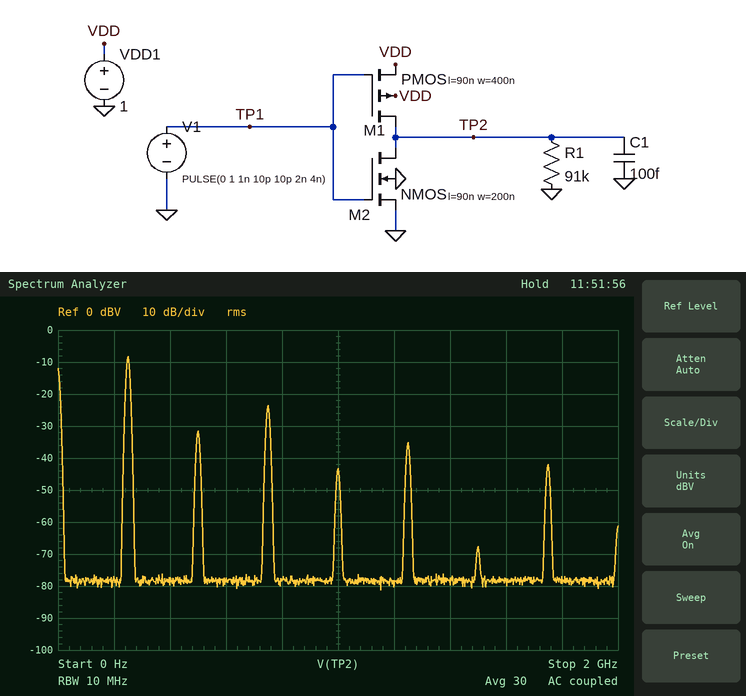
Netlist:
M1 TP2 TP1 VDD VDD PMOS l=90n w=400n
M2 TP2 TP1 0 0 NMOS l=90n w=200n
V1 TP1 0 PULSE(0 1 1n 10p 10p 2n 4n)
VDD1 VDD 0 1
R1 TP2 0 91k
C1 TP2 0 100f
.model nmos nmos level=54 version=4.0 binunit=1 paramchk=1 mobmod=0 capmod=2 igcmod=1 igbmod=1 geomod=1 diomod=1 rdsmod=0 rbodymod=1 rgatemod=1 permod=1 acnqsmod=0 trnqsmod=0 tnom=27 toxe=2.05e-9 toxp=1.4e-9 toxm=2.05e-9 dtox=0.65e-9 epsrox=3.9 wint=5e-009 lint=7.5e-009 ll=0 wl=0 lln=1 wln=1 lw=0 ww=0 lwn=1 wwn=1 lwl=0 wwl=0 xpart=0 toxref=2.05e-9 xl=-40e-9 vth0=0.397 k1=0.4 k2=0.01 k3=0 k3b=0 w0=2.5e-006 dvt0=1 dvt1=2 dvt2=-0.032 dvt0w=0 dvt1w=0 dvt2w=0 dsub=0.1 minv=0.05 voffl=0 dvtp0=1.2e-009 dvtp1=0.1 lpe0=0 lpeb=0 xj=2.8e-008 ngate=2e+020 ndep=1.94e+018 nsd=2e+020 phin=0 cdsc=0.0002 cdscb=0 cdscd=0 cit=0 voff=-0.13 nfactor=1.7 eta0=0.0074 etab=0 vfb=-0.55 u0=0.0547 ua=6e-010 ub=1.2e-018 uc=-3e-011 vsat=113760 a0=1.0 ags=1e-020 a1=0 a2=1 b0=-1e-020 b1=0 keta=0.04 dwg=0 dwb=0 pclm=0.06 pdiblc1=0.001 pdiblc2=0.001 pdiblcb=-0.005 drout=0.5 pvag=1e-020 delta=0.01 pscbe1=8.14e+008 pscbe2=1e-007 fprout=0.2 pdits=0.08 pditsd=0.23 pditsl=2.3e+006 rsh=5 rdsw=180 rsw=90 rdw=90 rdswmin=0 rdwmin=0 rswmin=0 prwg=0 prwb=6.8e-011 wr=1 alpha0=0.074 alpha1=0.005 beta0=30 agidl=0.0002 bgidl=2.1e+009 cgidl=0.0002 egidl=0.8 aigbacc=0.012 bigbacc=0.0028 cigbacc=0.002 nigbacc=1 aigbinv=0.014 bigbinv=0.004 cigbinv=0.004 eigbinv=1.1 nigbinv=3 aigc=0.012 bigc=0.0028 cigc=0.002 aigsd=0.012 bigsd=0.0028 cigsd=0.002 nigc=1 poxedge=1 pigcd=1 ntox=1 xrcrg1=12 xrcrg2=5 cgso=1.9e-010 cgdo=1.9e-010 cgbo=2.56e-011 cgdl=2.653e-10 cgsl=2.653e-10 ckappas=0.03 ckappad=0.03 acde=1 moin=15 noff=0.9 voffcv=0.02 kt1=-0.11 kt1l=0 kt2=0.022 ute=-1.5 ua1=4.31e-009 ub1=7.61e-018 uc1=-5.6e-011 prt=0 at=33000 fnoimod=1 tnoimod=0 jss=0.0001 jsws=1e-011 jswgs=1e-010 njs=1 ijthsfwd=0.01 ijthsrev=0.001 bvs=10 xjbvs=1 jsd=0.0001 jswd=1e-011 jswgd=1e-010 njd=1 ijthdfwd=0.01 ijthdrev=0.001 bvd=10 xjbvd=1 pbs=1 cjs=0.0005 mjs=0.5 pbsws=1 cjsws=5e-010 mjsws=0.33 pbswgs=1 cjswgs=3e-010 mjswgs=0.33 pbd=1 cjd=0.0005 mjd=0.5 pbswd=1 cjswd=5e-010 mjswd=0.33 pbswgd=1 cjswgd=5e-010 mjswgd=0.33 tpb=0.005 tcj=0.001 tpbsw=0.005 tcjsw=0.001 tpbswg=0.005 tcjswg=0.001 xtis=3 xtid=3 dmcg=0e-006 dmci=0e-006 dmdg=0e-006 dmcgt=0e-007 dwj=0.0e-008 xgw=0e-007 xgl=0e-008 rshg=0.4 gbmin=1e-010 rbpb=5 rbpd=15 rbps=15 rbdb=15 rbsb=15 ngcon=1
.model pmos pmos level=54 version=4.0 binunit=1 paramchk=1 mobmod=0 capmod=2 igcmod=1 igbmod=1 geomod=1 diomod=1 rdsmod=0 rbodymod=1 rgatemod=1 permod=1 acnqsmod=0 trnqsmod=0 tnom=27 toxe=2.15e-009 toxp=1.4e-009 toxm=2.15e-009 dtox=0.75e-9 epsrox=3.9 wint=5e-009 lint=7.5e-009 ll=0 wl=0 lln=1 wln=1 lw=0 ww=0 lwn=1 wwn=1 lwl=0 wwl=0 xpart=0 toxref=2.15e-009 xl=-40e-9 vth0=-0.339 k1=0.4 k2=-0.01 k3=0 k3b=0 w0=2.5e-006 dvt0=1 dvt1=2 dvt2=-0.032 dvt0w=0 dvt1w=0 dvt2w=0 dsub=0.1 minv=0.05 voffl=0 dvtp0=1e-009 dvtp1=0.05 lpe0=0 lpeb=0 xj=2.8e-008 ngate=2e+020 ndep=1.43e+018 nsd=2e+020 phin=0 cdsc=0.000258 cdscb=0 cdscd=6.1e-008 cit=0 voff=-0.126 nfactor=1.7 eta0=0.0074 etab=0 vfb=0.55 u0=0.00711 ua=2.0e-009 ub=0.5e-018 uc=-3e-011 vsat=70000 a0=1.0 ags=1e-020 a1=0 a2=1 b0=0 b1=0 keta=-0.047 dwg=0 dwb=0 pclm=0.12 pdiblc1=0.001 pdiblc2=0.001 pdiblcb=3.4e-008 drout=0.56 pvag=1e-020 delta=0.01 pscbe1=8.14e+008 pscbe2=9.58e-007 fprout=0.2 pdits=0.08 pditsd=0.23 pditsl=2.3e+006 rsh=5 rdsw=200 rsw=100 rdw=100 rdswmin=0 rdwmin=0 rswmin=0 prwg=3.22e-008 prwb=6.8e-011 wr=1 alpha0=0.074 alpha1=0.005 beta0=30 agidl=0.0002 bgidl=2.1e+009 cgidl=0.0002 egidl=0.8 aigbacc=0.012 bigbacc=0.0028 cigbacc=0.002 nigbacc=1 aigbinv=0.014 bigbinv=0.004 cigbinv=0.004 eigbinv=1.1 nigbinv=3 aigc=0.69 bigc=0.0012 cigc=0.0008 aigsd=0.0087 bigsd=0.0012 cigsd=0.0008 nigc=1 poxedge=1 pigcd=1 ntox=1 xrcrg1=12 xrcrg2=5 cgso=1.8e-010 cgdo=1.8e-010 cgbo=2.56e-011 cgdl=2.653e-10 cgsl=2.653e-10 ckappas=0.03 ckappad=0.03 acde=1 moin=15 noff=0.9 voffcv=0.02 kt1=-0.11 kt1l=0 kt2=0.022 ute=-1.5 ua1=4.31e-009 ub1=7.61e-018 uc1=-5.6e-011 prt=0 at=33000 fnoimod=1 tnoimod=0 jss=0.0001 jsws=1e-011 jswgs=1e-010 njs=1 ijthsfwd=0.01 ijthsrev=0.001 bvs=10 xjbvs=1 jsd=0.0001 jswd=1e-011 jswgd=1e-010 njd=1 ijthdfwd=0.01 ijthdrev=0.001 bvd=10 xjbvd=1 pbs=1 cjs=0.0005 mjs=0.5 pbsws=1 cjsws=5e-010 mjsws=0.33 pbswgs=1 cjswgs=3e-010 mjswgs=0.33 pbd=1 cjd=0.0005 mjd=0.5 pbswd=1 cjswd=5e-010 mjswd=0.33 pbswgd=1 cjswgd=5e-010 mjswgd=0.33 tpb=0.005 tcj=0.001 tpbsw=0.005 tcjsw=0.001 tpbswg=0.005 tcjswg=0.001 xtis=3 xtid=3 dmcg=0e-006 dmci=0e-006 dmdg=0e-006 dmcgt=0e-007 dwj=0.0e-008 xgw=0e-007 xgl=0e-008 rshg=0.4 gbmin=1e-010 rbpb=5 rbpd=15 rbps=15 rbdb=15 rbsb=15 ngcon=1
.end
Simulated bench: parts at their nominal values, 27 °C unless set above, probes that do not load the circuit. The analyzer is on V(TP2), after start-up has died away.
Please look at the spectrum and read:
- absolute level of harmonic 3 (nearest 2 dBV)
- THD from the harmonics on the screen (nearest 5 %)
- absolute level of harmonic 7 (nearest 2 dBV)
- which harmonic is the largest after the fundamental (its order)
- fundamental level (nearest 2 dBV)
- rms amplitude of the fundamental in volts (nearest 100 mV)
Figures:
-24 dBV
20 %
-42 dBV
3
-8 dBV
400 mV
